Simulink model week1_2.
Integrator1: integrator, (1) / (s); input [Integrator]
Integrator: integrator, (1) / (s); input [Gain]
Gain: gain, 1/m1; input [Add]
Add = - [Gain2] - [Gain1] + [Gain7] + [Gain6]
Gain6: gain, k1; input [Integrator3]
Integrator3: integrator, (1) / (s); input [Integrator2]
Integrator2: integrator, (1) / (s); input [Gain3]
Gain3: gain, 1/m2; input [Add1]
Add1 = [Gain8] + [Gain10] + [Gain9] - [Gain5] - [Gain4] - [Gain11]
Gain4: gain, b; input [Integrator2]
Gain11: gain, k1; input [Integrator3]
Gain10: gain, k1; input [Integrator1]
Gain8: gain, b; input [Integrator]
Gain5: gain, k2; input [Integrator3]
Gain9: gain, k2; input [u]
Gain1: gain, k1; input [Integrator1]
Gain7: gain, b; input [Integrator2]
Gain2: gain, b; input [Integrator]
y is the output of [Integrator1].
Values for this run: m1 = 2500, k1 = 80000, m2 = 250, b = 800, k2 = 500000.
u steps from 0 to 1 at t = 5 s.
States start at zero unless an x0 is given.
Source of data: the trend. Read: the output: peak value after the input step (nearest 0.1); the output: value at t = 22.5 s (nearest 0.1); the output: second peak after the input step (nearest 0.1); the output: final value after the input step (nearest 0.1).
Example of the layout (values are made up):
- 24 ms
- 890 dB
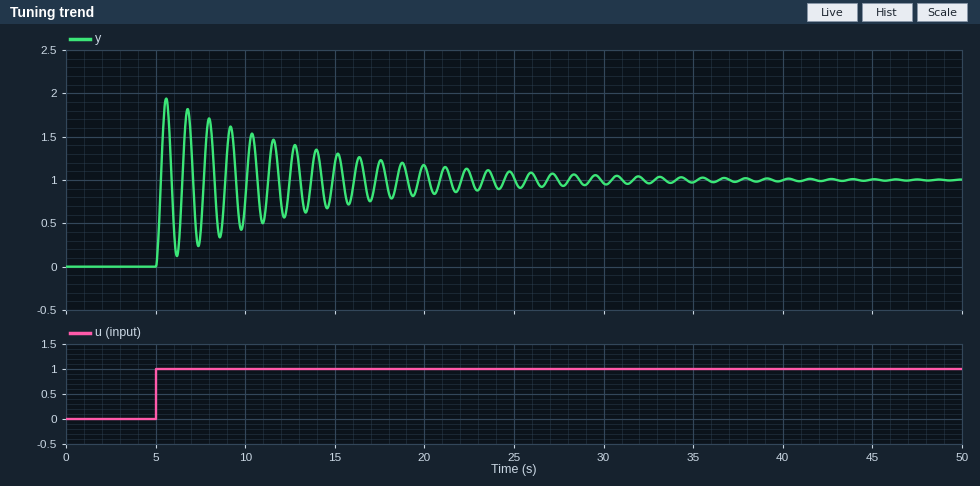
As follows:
- 1.9
- 1.1
- 1.8
- 1.0
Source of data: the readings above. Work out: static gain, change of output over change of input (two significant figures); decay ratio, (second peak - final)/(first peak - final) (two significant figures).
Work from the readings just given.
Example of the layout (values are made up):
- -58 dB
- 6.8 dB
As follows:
- 1.0
- 0.89
